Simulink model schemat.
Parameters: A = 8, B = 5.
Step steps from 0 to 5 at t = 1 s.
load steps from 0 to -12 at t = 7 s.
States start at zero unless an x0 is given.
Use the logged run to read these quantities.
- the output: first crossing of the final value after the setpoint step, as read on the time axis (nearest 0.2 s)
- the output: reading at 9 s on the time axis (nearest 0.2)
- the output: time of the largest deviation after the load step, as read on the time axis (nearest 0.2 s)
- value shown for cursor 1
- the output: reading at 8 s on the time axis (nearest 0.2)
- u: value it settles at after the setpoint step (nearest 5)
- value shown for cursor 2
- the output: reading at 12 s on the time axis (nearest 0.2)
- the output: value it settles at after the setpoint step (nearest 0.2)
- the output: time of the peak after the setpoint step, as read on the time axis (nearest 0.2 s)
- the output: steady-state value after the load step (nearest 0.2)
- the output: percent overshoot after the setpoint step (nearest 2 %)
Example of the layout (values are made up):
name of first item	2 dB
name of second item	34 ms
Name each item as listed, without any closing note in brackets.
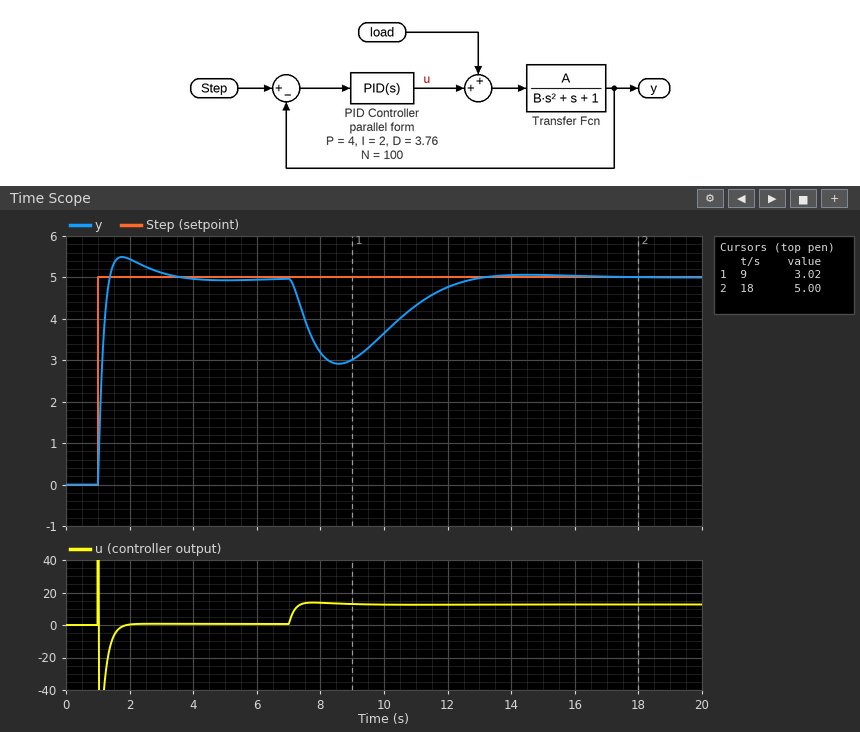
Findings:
the output: first crossing of the final value after the setpoint step, as read on the time axis	1.4 s
the output: reading at 9 s on the time axis	3.0
the output: time of the largest deviation after the load step, as read on the time axis	8.6 s
value shown for cursor 1	3.02
the output: reading at 8 s on the time axis	3.2
u: value it settles at after the setpoint step	0
value shown for cursor 2	5.00
the output: reading at 12 s on the time axis	4.8
the output: value it settles at after the setpoint step	5.0
the output: time of the peak after the setpoint step, as read on the time axis	1.8 s
the output: steady-state value after the load step	5.0
the output: percent overshoot after the setpoint step	10 %
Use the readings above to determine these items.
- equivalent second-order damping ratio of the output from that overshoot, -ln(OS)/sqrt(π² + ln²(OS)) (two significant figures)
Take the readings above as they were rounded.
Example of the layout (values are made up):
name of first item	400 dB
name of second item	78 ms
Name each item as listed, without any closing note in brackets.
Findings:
equivalent second-order damping ratio of the output from that overshoot, -ln(OS)/sqrt(π² + ln²(OS))	0.59
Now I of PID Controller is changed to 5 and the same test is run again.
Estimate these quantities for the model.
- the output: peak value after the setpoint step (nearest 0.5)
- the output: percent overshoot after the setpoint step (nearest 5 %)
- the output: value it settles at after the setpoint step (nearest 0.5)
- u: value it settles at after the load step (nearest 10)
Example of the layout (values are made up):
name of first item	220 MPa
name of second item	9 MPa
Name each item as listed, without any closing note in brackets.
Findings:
the output: peak value after the setpoint step	5.5
the output: percent overshoot after the setpoint step	15 %
the output: value it settles at after the setpoint step	5.0
u: value it settles at after the load step	10
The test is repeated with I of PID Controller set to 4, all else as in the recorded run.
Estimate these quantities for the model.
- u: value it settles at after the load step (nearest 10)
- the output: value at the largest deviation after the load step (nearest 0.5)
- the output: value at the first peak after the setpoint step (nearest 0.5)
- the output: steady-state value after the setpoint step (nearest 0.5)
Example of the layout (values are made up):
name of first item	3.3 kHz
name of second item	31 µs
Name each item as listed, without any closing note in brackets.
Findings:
u: value it settles at after the load step	10
the output: value at the largest deviation after the load step	3.0
the output: value at the first peak after the setpoint step	5.5
the output: steady-state value after the setpoint step	5.0
